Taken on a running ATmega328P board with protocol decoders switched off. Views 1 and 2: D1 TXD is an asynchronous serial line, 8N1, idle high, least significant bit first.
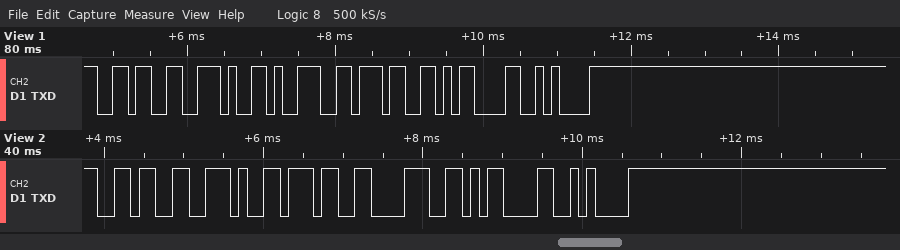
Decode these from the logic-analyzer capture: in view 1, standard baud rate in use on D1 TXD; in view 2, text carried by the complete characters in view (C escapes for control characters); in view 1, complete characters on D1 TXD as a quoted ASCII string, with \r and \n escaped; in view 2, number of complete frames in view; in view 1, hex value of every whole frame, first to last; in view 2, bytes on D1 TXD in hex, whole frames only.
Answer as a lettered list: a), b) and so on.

a) 9600 baud
b) "6.78\r\n"
c) "6.97\r\n"
d) 6
e) 0x36 0x2E 0x39 0x37 0x0D 0x0A
f) 36 2E 37 38 0D 0A
